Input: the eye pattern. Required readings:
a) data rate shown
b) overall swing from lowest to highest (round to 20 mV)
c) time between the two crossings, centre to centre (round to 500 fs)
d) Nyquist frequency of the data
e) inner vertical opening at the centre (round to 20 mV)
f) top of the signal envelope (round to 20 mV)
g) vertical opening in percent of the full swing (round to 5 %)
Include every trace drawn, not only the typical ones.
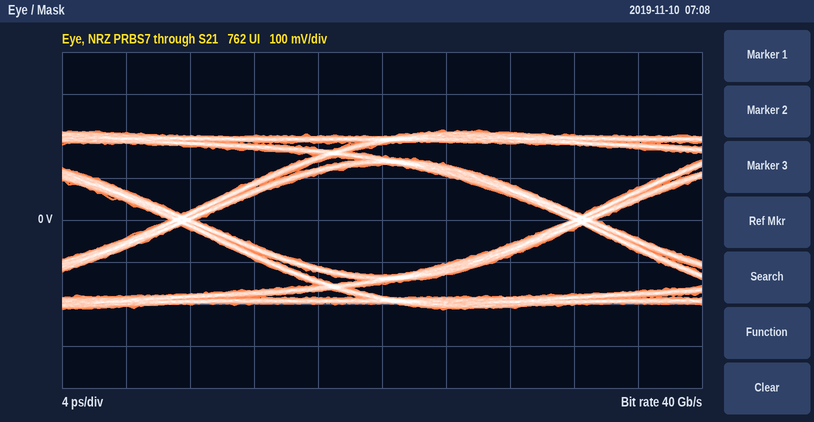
40 Gb/s
420 mV
25.0 ps
20 GHz
260 mV
220 mV
60 %
